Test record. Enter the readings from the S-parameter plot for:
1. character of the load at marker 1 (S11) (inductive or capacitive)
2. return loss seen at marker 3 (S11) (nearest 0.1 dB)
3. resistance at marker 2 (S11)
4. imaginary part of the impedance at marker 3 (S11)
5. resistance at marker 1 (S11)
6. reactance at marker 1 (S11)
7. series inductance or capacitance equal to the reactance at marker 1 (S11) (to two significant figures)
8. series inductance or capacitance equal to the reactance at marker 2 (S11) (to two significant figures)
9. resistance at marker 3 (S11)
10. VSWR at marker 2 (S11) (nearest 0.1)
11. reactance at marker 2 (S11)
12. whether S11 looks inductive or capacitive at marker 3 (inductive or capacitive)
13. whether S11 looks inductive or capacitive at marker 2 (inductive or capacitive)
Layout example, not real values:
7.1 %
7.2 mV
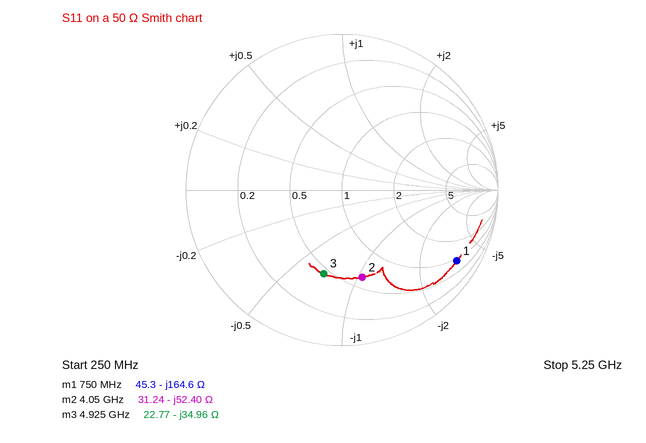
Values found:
capacitive
5.2 dB
31.24 Ω
-34.96 Ω
45.3 Ω
-164.6 Ω
1.3 pF
750 fF
22.77 Ω
3.7
-52.40 Ω
capacitive
capacitive
